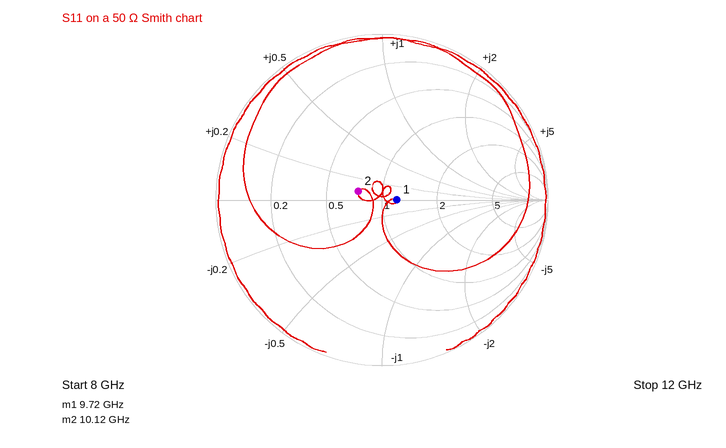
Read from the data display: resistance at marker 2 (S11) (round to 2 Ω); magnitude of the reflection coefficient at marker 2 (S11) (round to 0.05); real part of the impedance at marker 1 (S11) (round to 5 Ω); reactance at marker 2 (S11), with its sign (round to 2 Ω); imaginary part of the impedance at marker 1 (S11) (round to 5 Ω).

38 Ω
0.15
60 Ω
+4 Ω
0 Ω
